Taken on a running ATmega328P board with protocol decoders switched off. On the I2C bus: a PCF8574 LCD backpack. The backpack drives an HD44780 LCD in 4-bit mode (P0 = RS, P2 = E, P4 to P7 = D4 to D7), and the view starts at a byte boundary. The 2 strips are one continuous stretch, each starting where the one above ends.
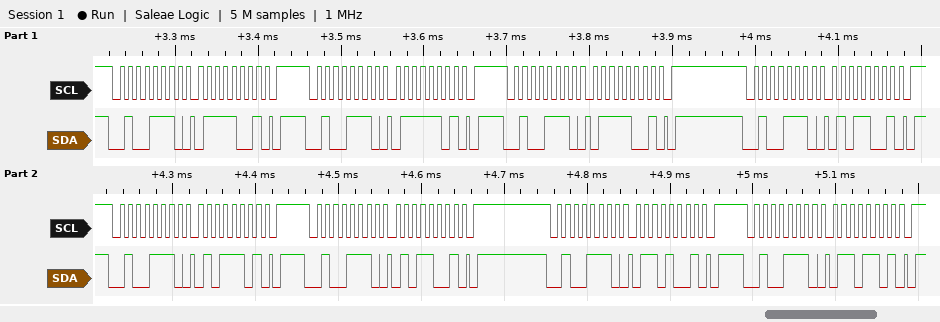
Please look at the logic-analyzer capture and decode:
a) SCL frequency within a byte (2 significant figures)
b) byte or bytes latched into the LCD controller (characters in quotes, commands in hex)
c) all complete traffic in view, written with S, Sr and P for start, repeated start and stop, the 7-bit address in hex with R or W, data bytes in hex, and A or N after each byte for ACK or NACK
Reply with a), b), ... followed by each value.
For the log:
a) 100 kHz
b) 'u'
c) S 27W A 79 A P S 27W A 7D A P S 27W A 79 A P S 27W A 59 A P S 27W A 5D A P S 27W A 59 A P S 27W A 69 A P S 27W A 6D A P
